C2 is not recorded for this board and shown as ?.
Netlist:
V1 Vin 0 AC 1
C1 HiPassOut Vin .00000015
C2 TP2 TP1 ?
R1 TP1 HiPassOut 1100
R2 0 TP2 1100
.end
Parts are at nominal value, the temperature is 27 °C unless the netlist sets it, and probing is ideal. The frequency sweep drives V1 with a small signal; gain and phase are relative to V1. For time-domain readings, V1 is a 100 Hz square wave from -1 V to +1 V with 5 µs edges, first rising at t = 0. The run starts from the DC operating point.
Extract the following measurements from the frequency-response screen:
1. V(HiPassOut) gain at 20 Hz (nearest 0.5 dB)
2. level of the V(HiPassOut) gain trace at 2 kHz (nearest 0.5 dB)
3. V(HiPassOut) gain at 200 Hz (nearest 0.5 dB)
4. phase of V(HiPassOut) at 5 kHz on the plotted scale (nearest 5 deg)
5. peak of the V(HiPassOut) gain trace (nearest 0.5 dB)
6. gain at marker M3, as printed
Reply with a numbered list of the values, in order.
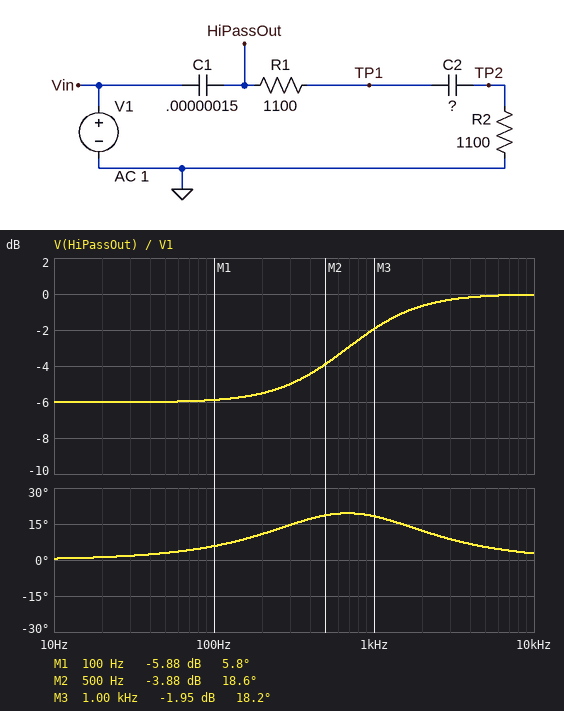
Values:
1. -6.0 dB
2. -0.5 dB
3. -5.5 dB
4. 5 deg
5. 0 dB
6. -1.95 dB
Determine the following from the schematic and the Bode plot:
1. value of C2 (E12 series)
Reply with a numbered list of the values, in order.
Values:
1. 150 nF
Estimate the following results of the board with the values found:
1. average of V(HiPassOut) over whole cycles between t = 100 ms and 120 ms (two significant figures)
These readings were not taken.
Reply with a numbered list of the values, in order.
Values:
1. 500 mV
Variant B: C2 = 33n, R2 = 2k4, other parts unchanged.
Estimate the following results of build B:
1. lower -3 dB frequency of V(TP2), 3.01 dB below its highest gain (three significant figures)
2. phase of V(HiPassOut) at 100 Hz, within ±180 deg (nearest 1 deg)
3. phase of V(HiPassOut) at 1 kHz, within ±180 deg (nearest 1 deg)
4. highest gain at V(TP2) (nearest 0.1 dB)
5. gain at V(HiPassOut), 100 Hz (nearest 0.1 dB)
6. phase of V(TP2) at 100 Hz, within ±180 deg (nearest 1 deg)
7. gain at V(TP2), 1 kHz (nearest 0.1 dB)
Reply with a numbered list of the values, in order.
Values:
1. 1.68 kHz
2. 1 deg
3. 5 deg
4. -3.3 dB
5. -1.7 dB
6. 87 deg
7. -9.1 dB
